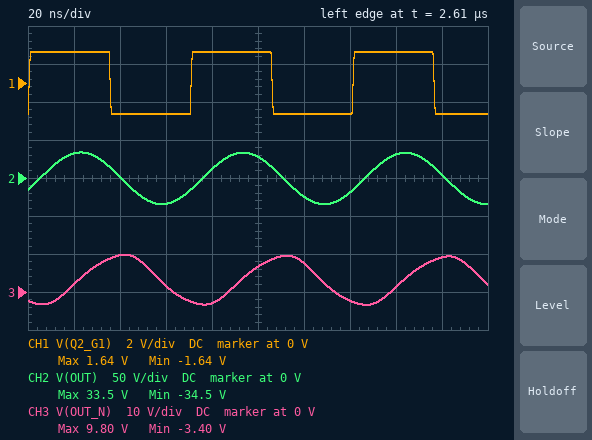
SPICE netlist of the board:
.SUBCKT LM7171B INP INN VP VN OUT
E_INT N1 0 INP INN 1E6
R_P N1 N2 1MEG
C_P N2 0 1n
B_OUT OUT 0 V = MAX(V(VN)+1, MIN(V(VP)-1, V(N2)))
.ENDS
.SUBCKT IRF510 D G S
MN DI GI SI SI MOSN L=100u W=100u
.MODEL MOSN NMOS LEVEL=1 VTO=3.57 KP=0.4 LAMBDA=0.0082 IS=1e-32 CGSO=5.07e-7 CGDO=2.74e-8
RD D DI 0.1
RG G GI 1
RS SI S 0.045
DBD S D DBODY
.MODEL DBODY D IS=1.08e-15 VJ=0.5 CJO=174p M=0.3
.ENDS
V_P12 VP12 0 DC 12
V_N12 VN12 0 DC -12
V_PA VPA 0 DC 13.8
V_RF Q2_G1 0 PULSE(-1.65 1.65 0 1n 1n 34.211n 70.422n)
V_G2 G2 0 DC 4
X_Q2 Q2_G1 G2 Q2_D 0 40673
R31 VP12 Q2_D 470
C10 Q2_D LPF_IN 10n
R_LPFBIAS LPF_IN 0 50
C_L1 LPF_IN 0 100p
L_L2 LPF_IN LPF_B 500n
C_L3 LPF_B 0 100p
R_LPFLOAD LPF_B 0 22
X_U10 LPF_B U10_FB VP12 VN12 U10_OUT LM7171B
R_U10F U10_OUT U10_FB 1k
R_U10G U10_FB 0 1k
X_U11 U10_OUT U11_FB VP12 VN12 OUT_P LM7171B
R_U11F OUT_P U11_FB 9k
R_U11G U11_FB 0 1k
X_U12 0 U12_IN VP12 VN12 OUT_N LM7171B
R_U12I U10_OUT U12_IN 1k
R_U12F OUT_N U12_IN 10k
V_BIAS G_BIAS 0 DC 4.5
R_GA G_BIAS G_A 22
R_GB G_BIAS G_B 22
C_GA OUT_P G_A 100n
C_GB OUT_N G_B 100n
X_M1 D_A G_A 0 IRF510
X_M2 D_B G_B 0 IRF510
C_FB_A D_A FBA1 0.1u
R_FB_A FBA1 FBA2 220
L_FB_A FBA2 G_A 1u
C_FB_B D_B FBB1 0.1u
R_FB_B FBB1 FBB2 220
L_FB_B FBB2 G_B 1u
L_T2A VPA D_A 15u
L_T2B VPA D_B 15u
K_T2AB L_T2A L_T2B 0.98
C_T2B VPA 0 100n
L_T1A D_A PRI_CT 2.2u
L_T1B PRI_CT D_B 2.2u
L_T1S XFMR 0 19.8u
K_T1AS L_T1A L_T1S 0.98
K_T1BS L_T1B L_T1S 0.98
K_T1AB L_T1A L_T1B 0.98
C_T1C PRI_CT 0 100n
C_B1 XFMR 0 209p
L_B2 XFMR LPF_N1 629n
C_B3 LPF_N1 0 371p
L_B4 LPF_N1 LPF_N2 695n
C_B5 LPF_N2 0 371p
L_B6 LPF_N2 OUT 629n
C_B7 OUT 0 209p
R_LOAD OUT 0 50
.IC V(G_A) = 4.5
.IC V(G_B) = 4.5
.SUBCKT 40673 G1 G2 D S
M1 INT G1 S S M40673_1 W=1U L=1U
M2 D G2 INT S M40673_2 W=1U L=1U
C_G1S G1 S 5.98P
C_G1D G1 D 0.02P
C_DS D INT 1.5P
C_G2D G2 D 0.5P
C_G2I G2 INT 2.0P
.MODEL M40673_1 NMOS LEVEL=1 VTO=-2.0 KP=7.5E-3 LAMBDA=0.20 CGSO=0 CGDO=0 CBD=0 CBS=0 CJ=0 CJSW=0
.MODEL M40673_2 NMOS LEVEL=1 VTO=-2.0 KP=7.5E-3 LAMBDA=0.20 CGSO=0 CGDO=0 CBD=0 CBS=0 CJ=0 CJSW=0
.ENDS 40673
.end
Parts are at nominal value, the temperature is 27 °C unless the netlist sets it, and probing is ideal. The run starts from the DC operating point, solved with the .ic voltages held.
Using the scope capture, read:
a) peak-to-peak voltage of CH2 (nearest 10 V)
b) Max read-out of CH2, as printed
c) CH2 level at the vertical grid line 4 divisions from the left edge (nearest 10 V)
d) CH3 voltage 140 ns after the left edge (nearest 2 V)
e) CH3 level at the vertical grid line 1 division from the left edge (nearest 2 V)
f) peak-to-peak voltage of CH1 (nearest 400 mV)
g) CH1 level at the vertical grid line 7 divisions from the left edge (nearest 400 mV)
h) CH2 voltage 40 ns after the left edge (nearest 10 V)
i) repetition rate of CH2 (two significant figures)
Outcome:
70 V
33.5 V
10 V
-2 V
2 V
3.2 V
-1.6 V
0 V
14 MHz
